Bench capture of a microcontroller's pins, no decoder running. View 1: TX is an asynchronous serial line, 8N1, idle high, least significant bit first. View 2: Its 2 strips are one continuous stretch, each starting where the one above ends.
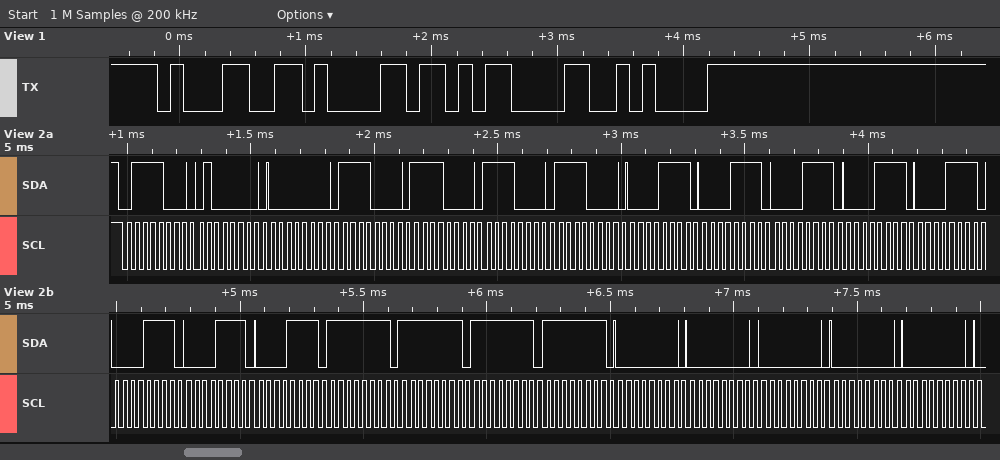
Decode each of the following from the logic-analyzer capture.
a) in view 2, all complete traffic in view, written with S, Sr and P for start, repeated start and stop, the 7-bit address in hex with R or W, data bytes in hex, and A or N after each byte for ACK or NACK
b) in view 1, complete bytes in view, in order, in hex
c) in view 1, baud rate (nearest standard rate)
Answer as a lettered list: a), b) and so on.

a) S 3CW A 40 A 00 A F0 A F0 A F0 A F0 A 0F A 0F A 0F A 0F A 0F A 0F A 0F A 0F A FF A FF A FF A FF A 00 A 00 A 00 A 00 A 00 A
b) 0x31 0x61 0x0D 0x0A
c) 9600 baud
